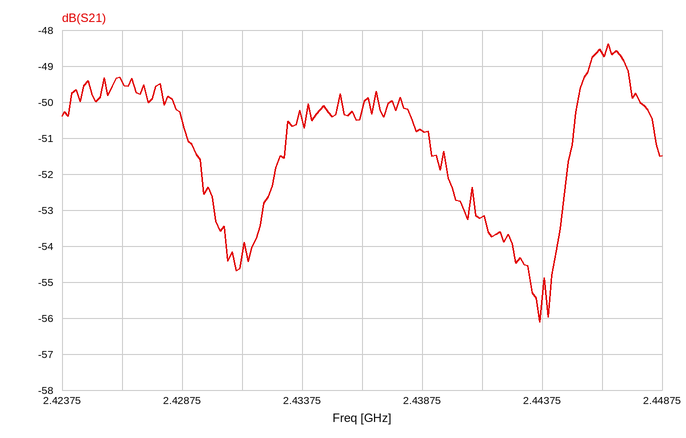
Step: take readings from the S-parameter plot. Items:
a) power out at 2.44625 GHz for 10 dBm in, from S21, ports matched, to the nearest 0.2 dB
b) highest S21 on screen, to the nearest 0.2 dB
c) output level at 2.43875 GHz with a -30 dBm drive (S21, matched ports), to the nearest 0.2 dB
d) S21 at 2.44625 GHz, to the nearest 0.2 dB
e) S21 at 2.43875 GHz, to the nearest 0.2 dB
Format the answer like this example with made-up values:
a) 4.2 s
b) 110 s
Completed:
a) -38.6 dBm
b) -48.4 dB
c) -80.8 dBm
d) -48.6 dB
e) -50.8 dB
